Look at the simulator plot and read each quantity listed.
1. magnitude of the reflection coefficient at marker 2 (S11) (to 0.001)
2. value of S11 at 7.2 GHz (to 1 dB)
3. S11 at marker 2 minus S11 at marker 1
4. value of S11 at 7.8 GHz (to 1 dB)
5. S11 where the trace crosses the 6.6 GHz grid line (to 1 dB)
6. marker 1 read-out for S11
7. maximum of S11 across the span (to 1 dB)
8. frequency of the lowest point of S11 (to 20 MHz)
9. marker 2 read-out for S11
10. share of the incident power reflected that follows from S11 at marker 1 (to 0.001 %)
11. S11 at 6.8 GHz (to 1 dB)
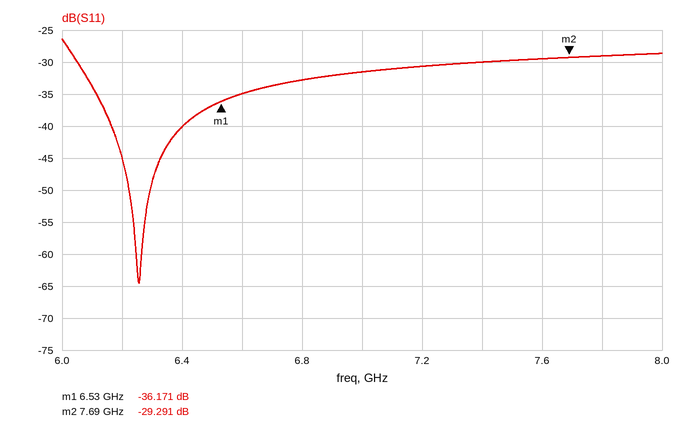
0.034
-31 dB
6.880 dB
-29 dB
-35 dB
-36.171 dB
-26 dB
6.26 GHz
-29.291 dB
0.024 %
-33 dB
